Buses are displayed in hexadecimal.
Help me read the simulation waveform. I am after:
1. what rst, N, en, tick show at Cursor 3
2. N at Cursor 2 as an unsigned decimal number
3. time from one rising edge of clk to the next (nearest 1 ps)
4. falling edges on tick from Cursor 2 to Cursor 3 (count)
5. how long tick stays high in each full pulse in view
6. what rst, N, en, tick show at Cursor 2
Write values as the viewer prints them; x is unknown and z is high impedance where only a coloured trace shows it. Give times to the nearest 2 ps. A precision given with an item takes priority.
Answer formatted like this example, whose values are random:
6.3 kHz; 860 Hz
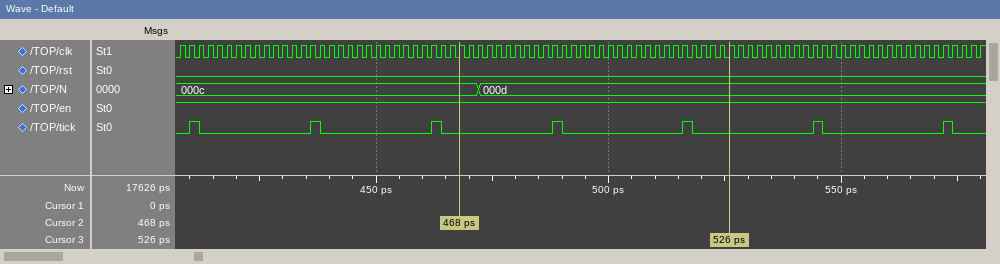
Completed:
rst=0, N=000d, en=1, tick=0; 12; 2 ps; 2; 2 ps, 2 ps, 2 ps, 2 ps, 2 ps, 2 ps, 2 ps; rst=0, N=000c, en=1, tick=0
